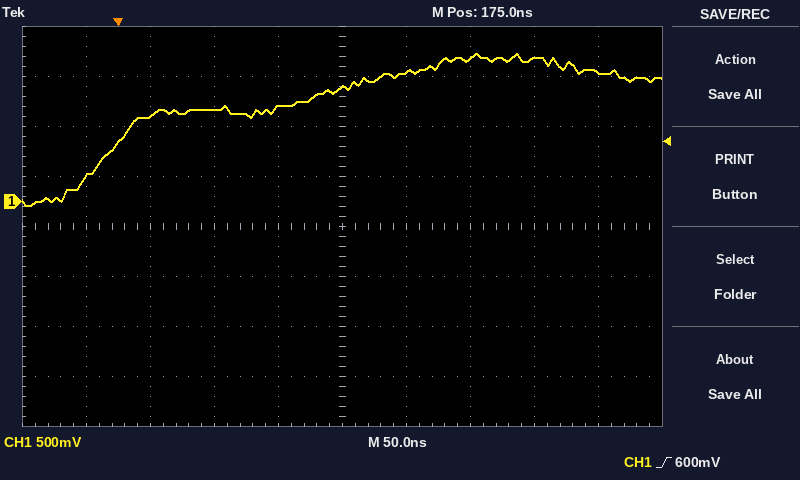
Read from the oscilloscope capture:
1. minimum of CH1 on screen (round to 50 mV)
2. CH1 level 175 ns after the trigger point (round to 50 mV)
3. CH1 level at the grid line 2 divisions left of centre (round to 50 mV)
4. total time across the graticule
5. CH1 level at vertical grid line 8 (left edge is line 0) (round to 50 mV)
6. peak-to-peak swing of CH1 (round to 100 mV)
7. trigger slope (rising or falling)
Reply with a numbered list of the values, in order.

1. -50 mV
2. 1.15 V
3. 900 mV
4. 500 ns
5. 1.45 V
6. 1.50 V
7. rising
